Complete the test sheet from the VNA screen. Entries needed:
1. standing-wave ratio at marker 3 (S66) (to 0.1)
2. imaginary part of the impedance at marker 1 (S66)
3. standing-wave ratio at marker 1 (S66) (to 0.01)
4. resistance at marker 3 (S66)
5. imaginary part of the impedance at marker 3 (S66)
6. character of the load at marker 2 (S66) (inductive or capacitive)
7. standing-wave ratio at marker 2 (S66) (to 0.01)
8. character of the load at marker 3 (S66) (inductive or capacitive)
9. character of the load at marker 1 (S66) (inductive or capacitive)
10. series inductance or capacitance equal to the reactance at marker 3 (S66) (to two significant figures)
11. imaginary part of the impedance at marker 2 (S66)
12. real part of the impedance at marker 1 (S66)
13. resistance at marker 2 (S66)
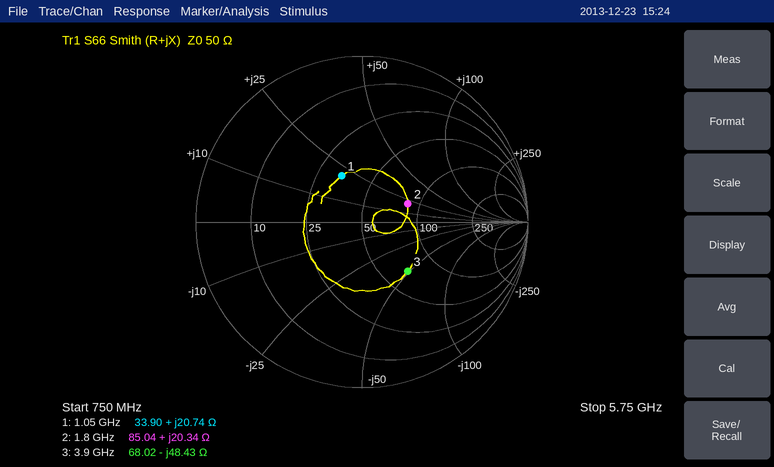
2.4
+20.74 Ω
1.87
68.02 Ω
-48.43 Ω
inductive
1.84
capacitive
inductive
840 fF
+20.34 Ω
33.90 Ω
85.04 Ω
